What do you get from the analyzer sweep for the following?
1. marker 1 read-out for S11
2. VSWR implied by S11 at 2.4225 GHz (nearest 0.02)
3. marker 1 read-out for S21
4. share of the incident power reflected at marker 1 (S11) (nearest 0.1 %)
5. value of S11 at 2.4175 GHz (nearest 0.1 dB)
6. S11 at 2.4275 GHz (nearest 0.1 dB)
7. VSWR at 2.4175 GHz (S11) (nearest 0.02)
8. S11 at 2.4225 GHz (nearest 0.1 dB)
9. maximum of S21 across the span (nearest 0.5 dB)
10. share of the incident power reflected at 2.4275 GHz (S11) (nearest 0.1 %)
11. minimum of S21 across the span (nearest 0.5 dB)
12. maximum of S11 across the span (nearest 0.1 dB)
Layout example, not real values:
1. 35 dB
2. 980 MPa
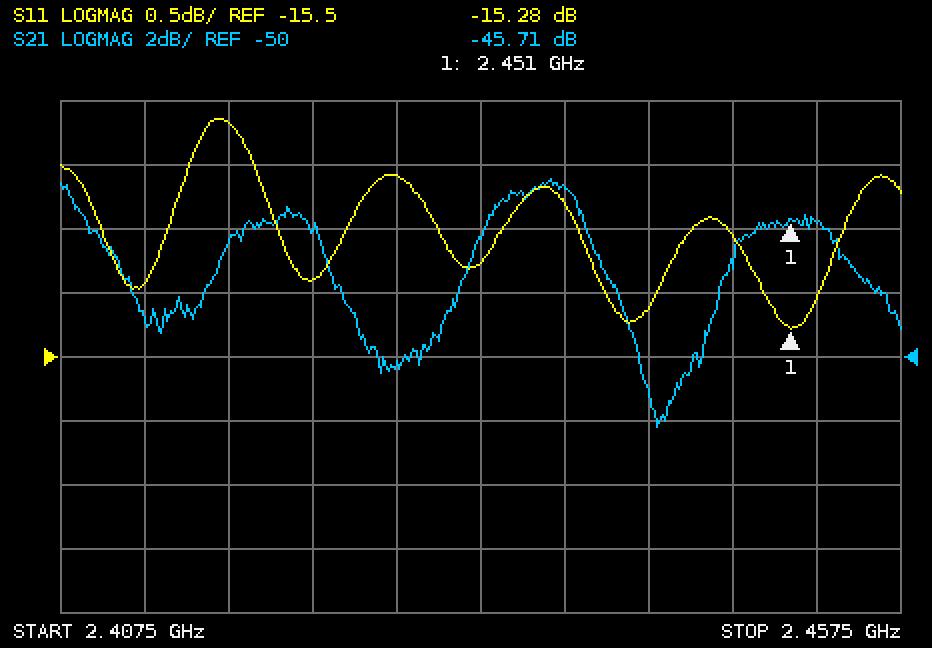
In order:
1. -15.28 dB
2. 1.44
3. -45.71 dB
4. 3.0 %
5. -13.7 dB
6. -14.1 dB
7. 1.52
8. -14.9 dB
9. -44.5 dB
10. 3.9 %
11. -52.0 dB
12. -13.6 dB
